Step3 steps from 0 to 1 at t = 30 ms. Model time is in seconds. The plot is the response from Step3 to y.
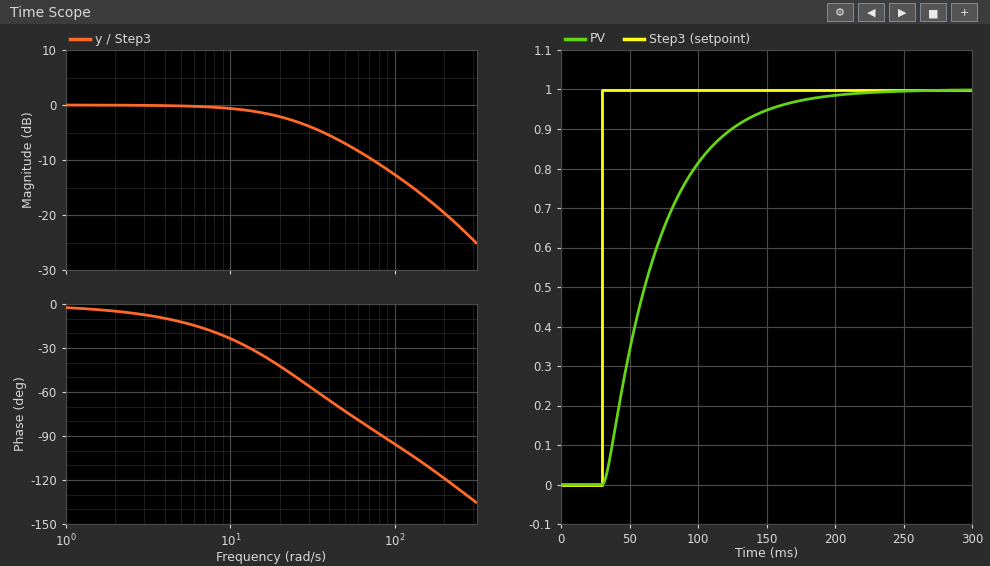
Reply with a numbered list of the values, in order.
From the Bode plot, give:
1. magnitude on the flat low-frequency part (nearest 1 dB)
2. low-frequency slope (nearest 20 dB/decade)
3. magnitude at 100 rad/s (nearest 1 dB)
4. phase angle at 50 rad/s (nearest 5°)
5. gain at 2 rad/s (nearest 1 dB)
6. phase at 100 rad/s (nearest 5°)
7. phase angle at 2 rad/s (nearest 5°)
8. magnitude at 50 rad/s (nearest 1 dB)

1. 0 dB
2. 0 dB/decade
3. -13 dB
4. -75°
5. 0 dB
6. -95°
7. -5°
8. -7 dB
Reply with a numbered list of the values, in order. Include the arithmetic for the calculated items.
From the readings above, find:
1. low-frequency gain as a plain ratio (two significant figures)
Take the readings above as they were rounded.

1. 10^(0 / 20) = 1.0
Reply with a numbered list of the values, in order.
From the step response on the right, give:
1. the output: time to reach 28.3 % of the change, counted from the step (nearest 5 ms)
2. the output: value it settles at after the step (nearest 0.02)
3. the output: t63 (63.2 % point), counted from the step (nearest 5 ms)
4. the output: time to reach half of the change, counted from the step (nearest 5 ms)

1. 15 ms
2. 1.00
3. 45 ms
4. 30 ms
